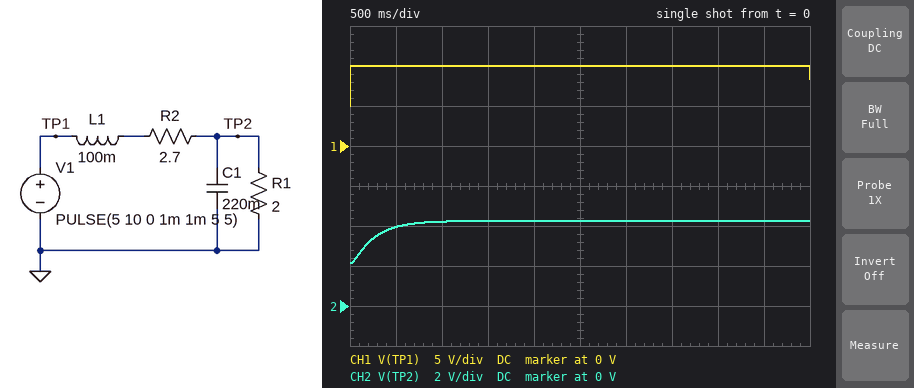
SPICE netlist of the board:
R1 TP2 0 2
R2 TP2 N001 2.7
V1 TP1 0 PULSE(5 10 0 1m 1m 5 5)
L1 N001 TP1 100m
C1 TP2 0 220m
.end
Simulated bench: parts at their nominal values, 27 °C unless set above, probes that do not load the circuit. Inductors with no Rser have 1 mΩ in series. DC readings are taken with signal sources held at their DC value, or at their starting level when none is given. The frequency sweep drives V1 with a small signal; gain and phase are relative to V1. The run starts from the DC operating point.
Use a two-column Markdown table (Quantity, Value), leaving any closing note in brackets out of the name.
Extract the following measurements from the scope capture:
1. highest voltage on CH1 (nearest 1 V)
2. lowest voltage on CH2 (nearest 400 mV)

| Quantity | Value |
|---|---|
| highest voltage on CH1 | 10 V |
| lowest voltage on CH2 | 2.0 V |
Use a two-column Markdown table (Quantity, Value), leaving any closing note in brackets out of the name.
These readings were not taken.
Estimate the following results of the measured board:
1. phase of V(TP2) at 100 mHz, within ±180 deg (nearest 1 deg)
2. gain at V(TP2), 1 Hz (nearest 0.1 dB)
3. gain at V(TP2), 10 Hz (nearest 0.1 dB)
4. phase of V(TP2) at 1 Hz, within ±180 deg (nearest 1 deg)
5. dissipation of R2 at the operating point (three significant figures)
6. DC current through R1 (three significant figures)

| Quantity | Value |
|---|---|
| phase of V(TP2) at 100 mHz, within ±180 deg | -10 deg |
| gain at V(TP2), 1 Hz | -12.7 dB |
| gain at V(TP2), 10 Hz | -39.4 dB |
| phase of V(TP2) at 1 Hz, within ±180 deg | -70 deg |
| dissipation of R2 at the operating point | 3.05 W |
| DC current through R1 | 1.06 A |
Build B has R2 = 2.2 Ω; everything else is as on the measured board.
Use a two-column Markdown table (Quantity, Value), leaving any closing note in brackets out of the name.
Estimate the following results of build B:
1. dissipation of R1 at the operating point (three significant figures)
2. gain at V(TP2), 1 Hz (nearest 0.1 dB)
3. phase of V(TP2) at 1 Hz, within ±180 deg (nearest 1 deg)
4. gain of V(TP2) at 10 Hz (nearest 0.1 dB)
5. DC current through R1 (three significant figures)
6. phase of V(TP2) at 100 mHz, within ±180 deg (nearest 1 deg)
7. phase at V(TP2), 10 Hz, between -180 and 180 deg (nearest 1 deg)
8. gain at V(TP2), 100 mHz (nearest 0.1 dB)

| Quantity | Value |
|---|---|
| dissipation of R1 at the operating point | 2.83 W |
| gain at V(TP2), 1 Hz | -11.1 dB |
| phase of V(TP2) at 1 Hz, within ±180 deg | -70 deg |
| gain of V(TP2) at 10 Hz | -39.2 dB |
| DC current through R1 | 1.19 A |
| phase of V(TP2) at 100 mHz, within ±180 deg | -9 deg |
| phase at V(TP2), 10 Hz, between -180 and 180 deg | -158 deg |
| gain at V(TP2), 100 mHz | -6.5 dB |
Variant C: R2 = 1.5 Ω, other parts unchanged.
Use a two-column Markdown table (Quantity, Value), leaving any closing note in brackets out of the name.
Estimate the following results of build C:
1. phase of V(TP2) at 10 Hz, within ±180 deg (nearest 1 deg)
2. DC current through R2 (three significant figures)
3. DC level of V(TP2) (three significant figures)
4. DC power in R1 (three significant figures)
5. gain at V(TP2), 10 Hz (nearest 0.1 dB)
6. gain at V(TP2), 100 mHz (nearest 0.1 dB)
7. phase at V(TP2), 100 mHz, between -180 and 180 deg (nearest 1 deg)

| Quantity | Value |
|---|---|
| phase of V(TP2) at 10 Hz, within ±180 deg | -164 deg |
| DC current through R2 | 1.43 A |
| DC level of V(TP2) | 2.86 V |
| DC power in R1 | 4.08 W |
| gain at V(TP2), 10 Hz | -38.9 dB |
| gain at V(TP2), 100 mHz | -4.9 dB |
| phase at V(TP2), 100 mHz, between -180 and 180 deg | -8 deg |
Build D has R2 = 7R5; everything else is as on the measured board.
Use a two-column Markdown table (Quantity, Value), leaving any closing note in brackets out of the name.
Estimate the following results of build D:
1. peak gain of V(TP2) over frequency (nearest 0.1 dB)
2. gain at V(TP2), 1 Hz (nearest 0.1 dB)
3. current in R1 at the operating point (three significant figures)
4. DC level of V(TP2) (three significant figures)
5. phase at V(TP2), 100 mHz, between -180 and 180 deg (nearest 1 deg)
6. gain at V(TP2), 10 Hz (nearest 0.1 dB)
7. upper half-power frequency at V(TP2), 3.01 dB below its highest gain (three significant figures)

| Quantity | Value |
|---|---|
| peak gain of V(TP2) over frequency | -13.5 dB |
| gain at V(TP2), 1 Hz | -21.1 dB |
| current in R1 at the operating point | 526 mA |
| DC level of V(TP2) | 1.05 V |
| phase at V(TP2), 100 mHz, between -180 and 180 deg | -13 deg |
| gain at V(TP2), 10 Hz | -42.6 dB |
| upper half-power frequency at V(TP2), 3.01 dB below its highest gain | 461 mHz |
